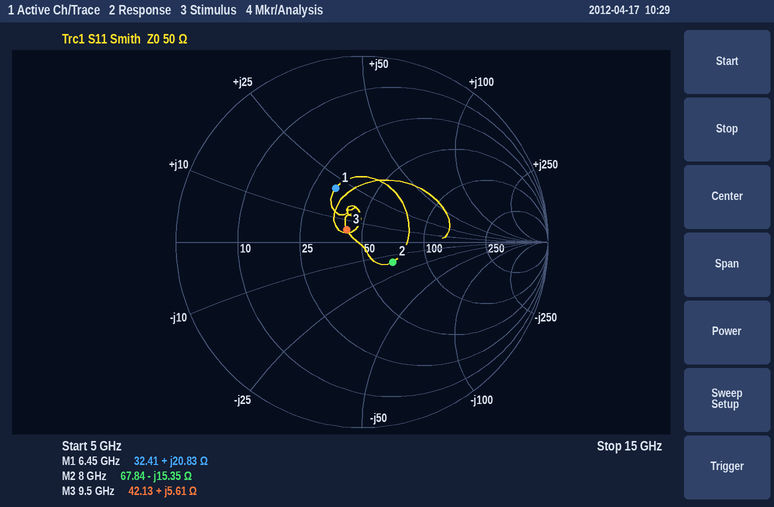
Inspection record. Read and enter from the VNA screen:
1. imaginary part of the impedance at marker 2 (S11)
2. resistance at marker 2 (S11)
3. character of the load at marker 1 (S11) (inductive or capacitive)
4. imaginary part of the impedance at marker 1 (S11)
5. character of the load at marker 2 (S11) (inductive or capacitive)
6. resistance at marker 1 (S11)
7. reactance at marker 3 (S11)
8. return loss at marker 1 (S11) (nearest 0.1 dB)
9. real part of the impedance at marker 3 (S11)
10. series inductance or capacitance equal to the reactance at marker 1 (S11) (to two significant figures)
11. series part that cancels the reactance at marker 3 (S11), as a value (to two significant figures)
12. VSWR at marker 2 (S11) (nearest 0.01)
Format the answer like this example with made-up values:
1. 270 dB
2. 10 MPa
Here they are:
1. -15.35 Ω
2. 67.84 Ω
3. inductive
4. +20.83 Ω
5. capacitive
6. 32.41 Ω
7. +5.61 Ω
8. 9.9 dB
9. 42.13 Ω
10. 510 pH
11. 3.0 pF
12. 1.49
